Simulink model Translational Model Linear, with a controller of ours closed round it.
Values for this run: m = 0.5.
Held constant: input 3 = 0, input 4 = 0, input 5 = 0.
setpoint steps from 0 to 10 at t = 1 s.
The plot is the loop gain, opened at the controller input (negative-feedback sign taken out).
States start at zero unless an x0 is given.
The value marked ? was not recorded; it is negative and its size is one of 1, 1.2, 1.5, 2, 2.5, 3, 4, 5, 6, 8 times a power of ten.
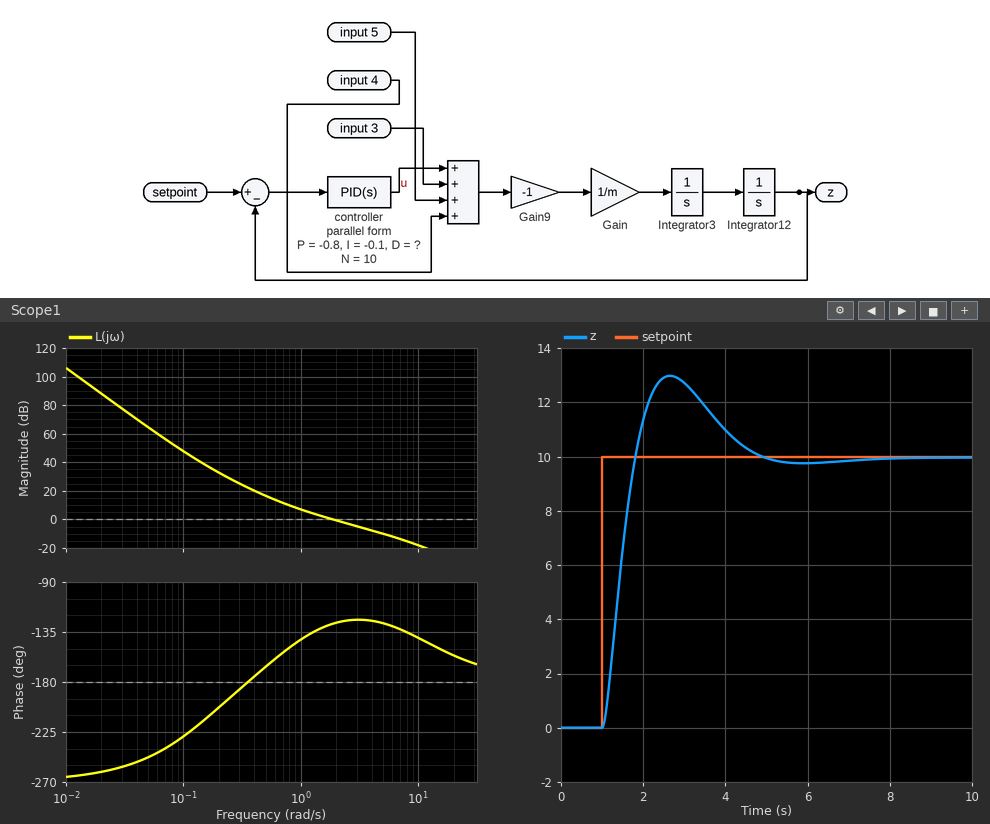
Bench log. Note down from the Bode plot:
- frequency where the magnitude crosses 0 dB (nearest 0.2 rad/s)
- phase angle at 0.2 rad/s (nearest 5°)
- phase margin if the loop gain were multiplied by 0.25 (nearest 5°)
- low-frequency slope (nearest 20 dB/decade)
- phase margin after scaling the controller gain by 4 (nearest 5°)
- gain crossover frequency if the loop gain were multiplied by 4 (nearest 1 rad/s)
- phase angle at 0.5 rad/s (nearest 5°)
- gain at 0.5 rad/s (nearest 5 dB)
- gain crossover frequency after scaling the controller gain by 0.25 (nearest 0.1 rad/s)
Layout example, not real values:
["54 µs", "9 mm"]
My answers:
["1.8 rad/s", "-205°", "25°", "-60 dB/decade", "50°", "6 rad/s", "-165°", "15 dB", "0.7 rad/s"]
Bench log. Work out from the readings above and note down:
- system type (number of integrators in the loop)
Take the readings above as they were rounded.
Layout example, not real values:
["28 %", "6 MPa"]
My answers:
["3"]
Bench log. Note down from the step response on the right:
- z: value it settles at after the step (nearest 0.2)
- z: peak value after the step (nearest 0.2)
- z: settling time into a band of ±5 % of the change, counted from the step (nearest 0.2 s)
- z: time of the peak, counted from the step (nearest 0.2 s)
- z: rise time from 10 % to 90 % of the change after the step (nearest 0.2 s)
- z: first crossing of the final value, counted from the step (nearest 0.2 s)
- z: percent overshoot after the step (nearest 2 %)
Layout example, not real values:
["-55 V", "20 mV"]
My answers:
["10.0", "13.0", "3.4 s", "1.6 s", "0.6 s", "0.8 s", "30 %"]
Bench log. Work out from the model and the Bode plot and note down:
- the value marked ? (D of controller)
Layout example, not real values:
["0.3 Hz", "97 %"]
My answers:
["-0.8"]
